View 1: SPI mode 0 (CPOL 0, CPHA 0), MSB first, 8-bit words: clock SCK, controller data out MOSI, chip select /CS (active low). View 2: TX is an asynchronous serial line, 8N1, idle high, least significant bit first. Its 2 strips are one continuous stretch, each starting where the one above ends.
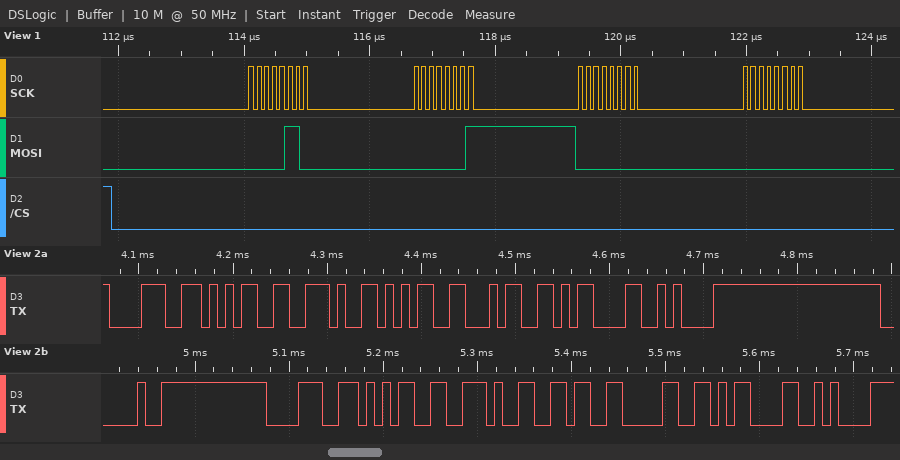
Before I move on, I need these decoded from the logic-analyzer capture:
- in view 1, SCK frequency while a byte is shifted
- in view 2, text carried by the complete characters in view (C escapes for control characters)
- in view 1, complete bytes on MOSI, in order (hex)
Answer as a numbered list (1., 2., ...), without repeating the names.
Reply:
1. 8 MHz
2. "85.54\r\n 85.60\r\n"
3. 06 01 00 00
